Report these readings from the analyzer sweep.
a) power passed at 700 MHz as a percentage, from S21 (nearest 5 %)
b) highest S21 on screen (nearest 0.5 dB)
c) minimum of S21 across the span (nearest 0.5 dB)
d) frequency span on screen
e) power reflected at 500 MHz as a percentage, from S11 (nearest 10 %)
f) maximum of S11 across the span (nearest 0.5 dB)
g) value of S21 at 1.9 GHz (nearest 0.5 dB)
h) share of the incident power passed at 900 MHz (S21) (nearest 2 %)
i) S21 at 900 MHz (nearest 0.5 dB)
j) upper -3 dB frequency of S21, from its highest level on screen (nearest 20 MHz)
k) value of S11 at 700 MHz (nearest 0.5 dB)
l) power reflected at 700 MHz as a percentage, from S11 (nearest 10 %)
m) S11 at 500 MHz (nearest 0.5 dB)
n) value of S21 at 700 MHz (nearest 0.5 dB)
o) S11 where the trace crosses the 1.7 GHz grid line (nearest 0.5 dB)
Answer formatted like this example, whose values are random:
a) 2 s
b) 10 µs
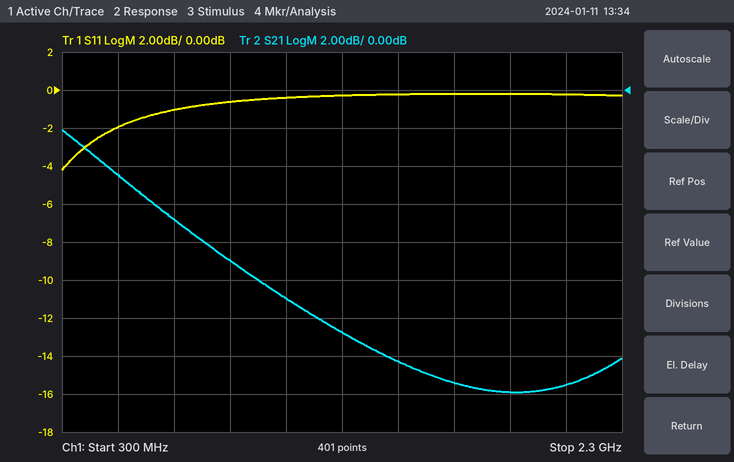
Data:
a) 20 %
b) -2.0 dB
c) -16.0 dB
d) 2 GHz
e) 60 %
f) 0.0 dB
g) -16.0 dB
h) 12 %
i) -9.0 dB
j) 560 MHz
k) -1.0 dB
l) 80 %
m) -2.0 dB
n) -7.0 dB
o) 0.0 dB
